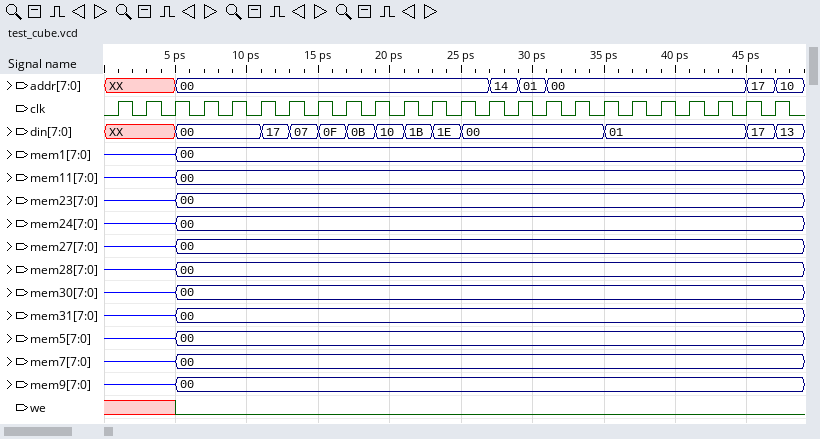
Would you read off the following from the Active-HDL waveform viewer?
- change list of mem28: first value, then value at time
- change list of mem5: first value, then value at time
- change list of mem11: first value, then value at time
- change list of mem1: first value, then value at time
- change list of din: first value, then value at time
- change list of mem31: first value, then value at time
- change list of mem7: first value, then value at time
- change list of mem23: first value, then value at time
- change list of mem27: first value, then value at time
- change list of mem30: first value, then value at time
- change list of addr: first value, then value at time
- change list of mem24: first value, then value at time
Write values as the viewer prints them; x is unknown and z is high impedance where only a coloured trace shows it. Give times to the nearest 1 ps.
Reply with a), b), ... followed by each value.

a) z, 00 at 5 ps
b) z, 00 at 5 ps
c) z, 00 at 5 ps
d) z, 00 at 5 ps
e) XX, 00 at 5 ps, 17 at 11 ps, 07 at 13 ps, 0F at 15 ps, 0B at 17 ps, 10 at 19 ps, 1B at 21 ps, 1E at 23 ps, 00 at 25 ps, 01 at 35 ps, 17 at 45 ps, 13 at 47 ps
f) z, 00 at 5 ps
g) z, 00 at 5 ps
h) z, 00 at 5 ps
i) z, 00 at 5 ps
j) z, 00 at 5 ps
k) XX, 00 at 5 ps, 14 at 27 ps, 01 at 29 ps, 00 at 31 ps, 17 at 45 ps, 10 at 47 ps
l) z, 00 at 5 ps
